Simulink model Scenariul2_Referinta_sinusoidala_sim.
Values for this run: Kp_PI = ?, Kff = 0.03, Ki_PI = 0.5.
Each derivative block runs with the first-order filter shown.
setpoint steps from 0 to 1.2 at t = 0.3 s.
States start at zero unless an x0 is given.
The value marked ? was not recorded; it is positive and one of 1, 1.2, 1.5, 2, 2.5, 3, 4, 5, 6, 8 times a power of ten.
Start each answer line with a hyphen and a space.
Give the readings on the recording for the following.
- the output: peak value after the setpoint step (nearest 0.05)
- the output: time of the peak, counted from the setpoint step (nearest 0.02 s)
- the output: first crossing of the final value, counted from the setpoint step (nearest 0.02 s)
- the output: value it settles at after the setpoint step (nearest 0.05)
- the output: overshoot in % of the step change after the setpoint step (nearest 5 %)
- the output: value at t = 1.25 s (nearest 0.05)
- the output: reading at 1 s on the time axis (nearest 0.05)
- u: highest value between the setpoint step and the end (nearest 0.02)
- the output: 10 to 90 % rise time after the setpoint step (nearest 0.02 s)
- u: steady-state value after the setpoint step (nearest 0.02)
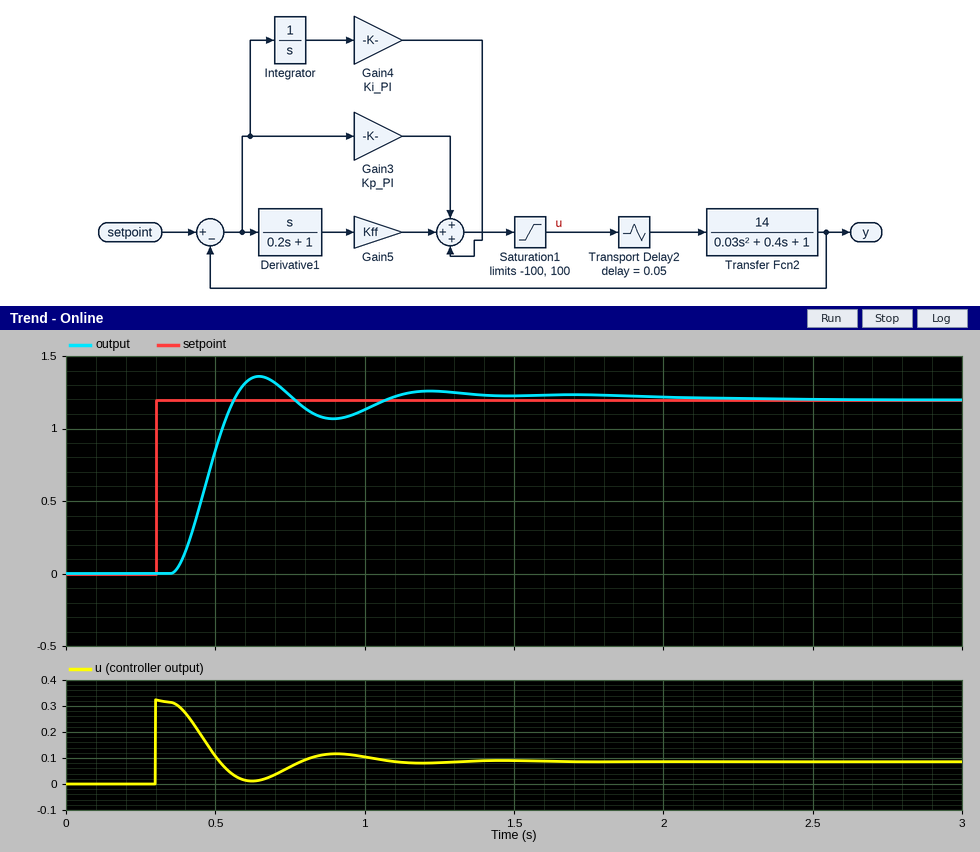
- 1.35
- 0.34 s
- 0.26 s
- 1.20
- 15 %
- 1.25
- 1.15
- 0.32
- 0.14 s
- 0.08
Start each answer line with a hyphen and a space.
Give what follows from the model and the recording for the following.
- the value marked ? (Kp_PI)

- 0.12
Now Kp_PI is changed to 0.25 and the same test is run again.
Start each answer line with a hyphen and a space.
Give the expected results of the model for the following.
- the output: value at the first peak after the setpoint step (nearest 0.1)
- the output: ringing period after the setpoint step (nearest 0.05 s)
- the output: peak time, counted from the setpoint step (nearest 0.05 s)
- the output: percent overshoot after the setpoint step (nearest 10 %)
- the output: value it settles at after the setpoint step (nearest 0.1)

- 1.7
- 0.50 s
- 0.30 s
- 40 %
- 1.2
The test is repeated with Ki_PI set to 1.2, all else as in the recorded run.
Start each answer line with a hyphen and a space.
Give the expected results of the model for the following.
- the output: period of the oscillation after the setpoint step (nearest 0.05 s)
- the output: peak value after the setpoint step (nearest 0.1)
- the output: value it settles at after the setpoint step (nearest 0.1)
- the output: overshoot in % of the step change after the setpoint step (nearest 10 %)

- 0.65 s
- 1.8
- 1.2
- 50 %
